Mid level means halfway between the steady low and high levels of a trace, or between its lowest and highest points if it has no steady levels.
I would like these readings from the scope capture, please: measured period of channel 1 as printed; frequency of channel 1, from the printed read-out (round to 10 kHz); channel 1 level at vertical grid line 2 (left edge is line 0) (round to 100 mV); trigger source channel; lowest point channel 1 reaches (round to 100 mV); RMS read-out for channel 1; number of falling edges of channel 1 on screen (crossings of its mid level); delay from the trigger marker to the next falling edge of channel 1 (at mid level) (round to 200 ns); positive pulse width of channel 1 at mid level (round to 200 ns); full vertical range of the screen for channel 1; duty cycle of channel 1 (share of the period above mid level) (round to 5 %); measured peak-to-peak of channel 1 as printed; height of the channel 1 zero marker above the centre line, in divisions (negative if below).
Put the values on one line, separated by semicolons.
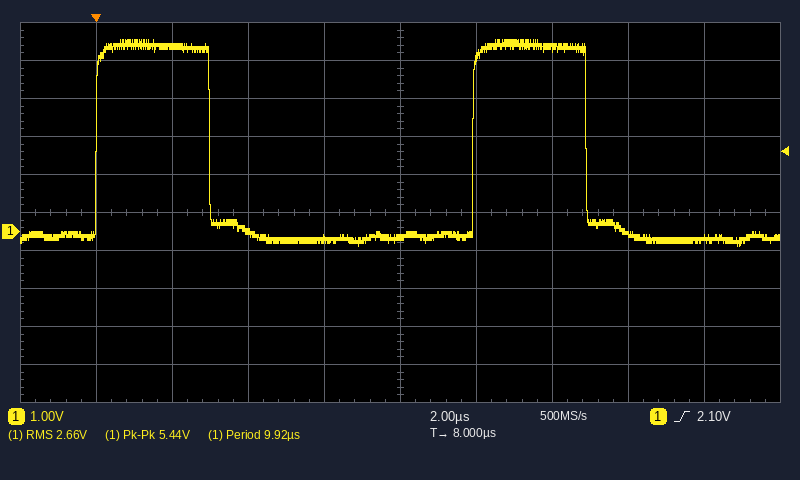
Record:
9.92 µs; 100 kHz; 4.9 V; channel 1; -400 mV; 2.66 V; 2; 3.0 µs; 3.0 µs; 10 V; 30 %; 5.44 V; -0.5 div
